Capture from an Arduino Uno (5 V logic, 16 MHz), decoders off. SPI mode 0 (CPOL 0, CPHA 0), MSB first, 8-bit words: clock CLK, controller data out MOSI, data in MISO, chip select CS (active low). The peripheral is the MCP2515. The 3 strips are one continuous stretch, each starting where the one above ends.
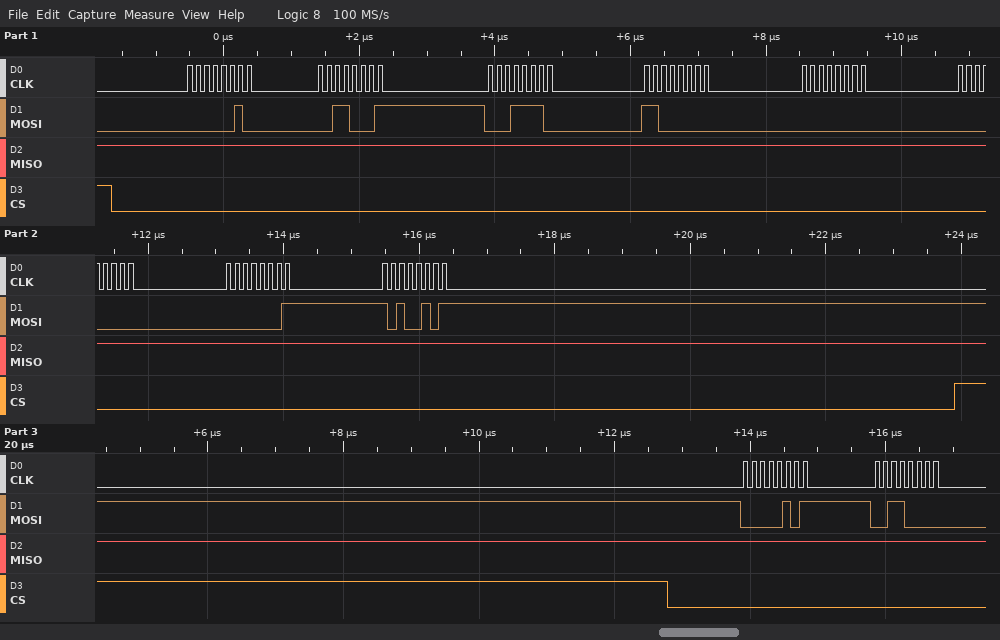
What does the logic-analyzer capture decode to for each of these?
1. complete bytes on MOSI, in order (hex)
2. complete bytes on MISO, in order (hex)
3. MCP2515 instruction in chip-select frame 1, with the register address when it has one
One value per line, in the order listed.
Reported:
02 31 1E C0 00 00 01 A5 05 30
FF FF FF FF FF FF FF FF FF FF
WRITE 0x31
